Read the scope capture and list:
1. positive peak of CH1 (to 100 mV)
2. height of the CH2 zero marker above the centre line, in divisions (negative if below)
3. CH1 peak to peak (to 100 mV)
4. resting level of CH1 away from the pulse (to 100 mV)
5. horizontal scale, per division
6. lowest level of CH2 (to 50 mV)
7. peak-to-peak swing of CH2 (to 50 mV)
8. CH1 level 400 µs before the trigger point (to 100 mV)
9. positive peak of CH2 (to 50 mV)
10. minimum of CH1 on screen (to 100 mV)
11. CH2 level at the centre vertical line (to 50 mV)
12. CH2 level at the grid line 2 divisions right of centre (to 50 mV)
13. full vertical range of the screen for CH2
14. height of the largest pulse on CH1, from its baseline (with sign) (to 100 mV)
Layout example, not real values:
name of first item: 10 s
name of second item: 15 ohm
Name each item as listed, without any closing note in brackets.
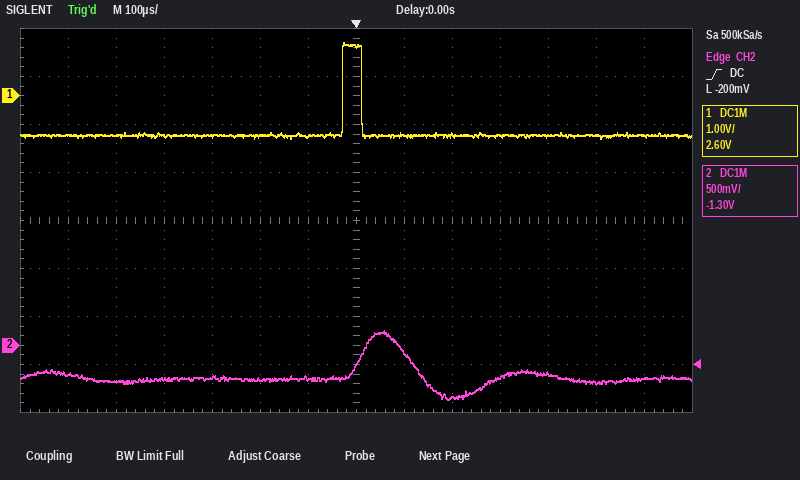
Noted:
positive peak of CH1: 1.1 V
height of the CH2 zero marker above the centre line, in divisions: -2.6 div
CH1 peak to peak: 2.0 V
resting level of CH1 away from the pulse: -800 mV
horizontal scale, per division: 100 µs
lowest level of CH2: -550 mV
peak-to-peak swing of CH2: 700 mV
CH1 level 400 µs before the trigger point: -800 mV
positive peak of CH2: 150 mV
minimum of CH1 on screen: -900 mV
CH2 level at the centre vertical line: -200 mV
CH2 level at the grid line 2 divisions right of centre: -550 mV
full vertical range of the screen for CH2: 4 V
height of the largest pulse on CH1, from its baseline (with sign): +1.9 V
